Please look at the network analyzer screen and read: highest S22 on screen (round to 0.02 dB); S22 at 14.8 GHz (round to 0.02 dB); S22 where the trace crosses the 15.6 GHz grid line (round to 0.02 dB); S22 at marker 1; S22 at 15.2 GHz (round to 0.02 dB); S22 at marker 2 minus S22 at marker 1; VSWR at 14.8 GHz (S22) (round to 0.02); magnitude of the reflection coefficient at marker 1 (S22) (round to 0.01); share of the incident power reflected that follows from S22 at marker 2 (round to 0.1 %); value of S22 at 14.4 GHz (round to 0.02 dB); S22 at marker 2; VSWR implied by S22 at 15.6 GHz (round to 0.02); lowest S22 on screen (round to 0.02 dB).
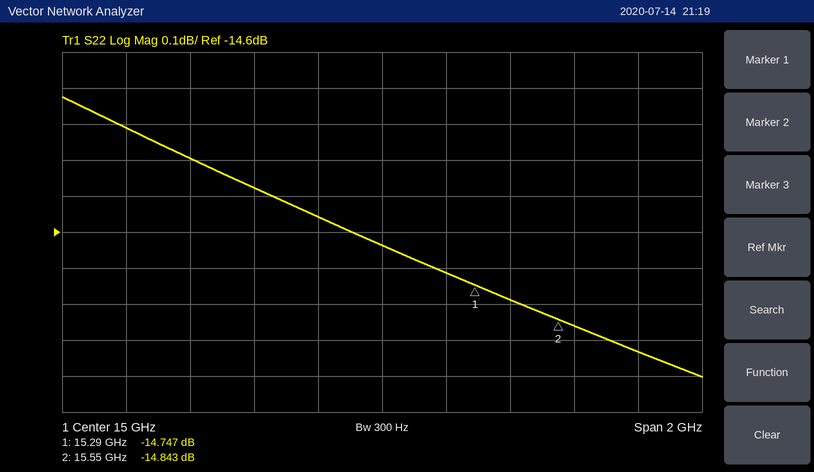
-14.22 dB
-14.56 dB
-14.86 dB
-14.747 dB
-14.72 dB
-0.096 dB
1.46
0.18
3.3 %
-14.40 dB
-14.843 dB
1.44
-15.00 dB
